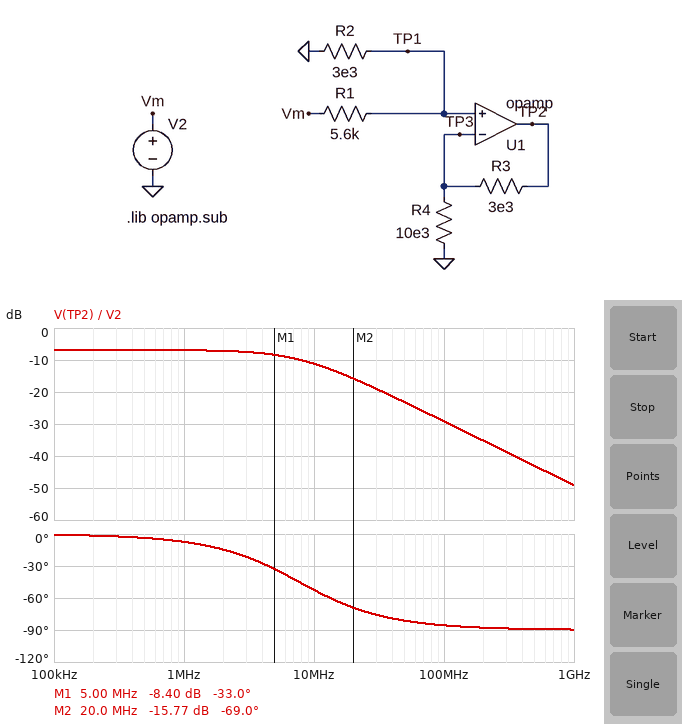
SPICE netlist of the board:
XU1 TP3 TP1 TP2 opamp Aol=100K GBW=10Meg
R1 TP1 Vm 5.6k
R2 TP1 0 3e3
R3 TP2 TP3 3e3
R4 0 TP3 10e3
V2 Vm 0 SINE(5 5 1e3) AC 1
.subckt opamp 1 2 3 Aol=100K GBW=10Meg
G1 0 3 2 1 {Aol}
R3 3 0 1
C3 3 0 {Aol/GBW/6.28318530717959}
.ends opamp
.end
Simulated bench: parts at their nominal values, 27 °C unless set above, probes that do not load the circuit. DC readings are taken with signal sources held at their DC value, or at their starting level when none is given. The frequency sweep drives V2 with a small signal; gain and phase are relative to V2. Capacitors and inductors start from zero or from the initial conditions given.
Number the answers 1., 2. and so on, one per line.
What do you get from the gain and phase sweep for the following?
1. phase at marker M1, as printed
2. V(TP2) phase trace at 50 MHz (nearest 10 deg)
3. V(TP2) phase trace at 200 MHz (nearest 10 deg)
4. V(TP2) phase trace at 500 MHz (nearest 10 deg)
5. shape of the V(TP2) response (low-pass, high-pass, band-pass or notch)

1. -33.0 deg
2. -80 deg
3. -90 deg
4. -90 deg
5. low-pass
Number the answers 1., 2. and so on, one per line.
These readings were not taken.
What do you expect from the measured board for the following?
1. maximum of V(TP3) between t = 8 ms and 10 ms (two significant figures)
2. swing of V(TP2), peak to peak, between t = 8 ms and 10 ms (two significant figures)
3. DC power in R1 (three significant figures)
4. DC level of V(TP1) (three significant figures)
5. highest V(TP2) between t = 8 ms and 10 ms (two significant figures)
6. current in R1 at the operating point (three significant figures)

1. 3.5 V
2. 4.5 V
3. 1.89 mW
4. 1.74 V
5. 4.5 V
6. 581 µA
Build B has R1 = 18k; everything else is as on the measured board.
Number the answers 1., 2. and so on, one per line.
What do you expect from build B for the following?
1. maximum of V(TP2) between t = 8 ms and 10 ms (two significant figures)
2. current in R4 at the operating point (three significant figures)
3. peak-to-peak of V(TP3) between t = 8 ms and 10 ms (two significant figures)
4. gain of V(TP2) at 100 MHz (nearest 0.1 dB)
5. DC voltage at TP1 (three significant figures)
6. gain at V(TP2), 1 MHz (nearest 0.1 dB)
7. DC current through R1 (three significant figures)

1. 1.9 V
2. 71.4 µA
3. 1.4 V
4. -36.9 dB
5. 714 mV
6. -14.7 dB
7. 238 µA
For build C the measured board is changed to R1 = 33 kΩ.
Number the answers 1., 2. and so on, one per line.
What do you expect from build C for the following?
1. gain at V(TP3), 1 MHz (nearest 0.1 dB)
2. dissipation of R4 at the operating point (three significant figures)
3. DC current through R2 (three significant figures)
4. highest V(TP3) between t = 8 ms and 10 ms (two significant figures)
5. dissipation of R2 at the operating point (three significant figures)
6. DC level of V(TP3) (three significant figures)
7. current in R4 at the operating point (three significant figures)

1. -21.7 dB
2. 17.4 µW
3. 139 µA
4. 830 mV
5. 57.9 µW
6. 417 mV
7. 41.7 µA
